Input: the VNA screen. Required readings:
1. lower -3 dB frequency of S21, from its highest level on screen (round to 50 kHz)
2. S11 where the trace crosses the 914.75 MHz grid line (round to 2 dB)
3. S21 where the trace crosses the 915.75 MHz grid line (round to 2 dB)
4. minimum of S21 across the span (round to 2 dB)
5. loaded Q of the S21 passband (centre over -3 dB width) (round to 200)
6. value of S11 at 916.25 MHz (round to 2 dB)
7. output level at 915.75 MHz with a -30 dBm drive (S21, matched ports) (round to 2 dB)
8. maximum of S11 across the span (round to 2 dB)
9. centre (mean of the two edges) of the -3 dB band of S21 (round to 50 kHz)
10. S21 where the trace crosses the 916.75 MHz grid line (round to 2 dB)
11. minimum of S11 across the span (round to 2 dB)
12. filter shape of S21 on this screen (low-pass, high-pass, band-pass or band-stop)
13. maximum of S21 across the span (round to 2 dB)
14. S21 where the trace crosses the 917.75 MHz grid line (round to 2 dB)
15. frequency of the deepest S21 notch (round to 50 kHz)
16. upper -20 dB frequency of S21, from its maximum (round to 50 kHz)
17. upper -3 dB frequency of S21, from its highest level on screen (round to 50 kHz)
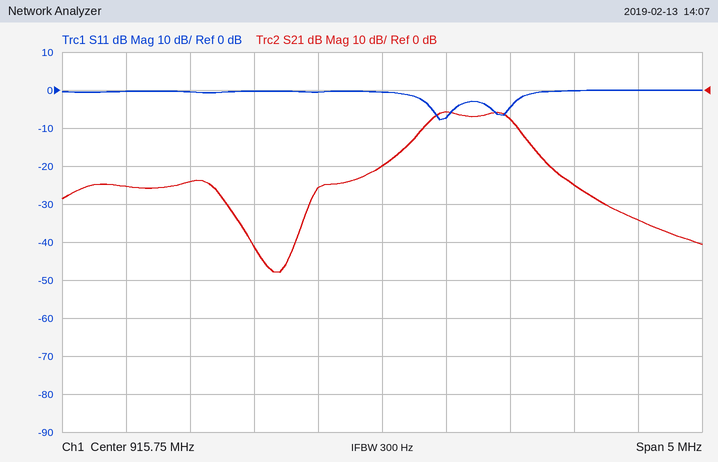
916.10 MHz
0 dB
-20 dB
-48 dB
1400
-8 dB
-50 dBm
0 dB
916.45 MHz
-8 dB
-8 dB
band-pass
-6 dB
-34 dB
914.95 MHz
917.30 MHz
916.80 MHz
